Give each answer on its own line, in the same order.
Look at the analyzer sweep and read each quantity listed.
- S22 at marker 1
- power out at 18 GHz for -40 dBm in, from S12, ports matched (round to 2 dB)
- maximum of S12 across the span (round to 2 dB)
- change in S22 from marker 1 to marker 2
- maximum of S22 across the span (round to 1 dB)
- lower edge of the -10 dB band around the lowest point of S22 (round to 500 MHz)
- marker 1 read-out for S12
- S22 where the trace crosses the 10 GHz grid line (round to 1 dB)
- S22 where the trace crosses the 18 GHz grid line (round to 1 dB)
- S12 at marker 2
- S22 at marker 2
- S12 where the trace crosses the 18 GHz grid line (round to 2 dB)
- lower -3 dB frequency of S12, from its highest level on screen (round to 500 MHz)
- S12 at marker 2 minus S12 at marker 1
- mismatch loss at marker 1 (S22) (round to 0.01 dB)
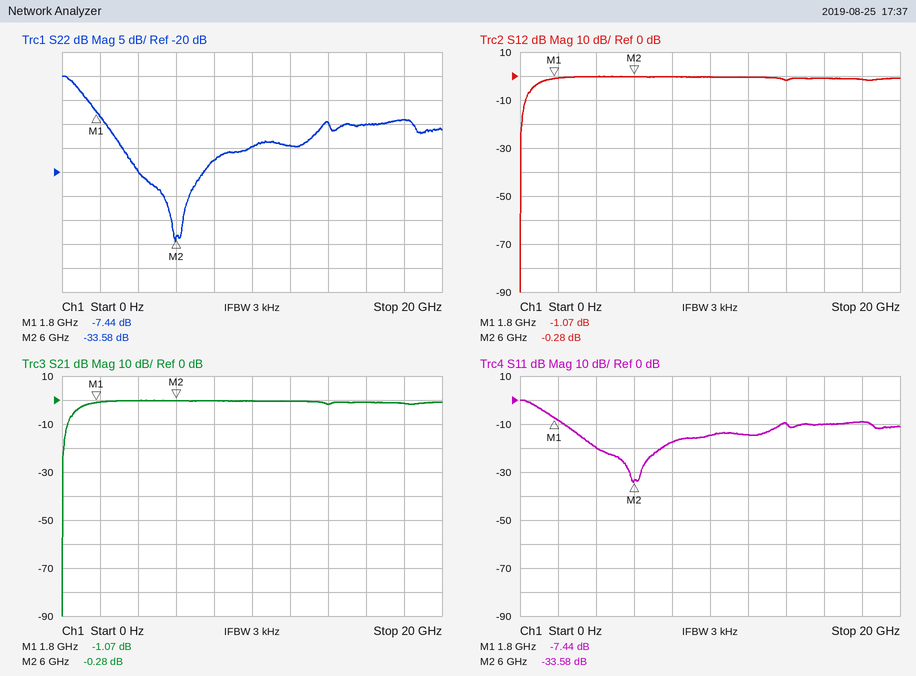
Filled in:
-7.44 dB
-42 dBm
0 dB
-26.14 dB
0 dB
2.5 GHz
-1.07 dB
-15 dB
-9 dB
-0.28 dB
-33.58 dB
-2 dB
1.0 GHz
0.79 dB
0.86 dB
